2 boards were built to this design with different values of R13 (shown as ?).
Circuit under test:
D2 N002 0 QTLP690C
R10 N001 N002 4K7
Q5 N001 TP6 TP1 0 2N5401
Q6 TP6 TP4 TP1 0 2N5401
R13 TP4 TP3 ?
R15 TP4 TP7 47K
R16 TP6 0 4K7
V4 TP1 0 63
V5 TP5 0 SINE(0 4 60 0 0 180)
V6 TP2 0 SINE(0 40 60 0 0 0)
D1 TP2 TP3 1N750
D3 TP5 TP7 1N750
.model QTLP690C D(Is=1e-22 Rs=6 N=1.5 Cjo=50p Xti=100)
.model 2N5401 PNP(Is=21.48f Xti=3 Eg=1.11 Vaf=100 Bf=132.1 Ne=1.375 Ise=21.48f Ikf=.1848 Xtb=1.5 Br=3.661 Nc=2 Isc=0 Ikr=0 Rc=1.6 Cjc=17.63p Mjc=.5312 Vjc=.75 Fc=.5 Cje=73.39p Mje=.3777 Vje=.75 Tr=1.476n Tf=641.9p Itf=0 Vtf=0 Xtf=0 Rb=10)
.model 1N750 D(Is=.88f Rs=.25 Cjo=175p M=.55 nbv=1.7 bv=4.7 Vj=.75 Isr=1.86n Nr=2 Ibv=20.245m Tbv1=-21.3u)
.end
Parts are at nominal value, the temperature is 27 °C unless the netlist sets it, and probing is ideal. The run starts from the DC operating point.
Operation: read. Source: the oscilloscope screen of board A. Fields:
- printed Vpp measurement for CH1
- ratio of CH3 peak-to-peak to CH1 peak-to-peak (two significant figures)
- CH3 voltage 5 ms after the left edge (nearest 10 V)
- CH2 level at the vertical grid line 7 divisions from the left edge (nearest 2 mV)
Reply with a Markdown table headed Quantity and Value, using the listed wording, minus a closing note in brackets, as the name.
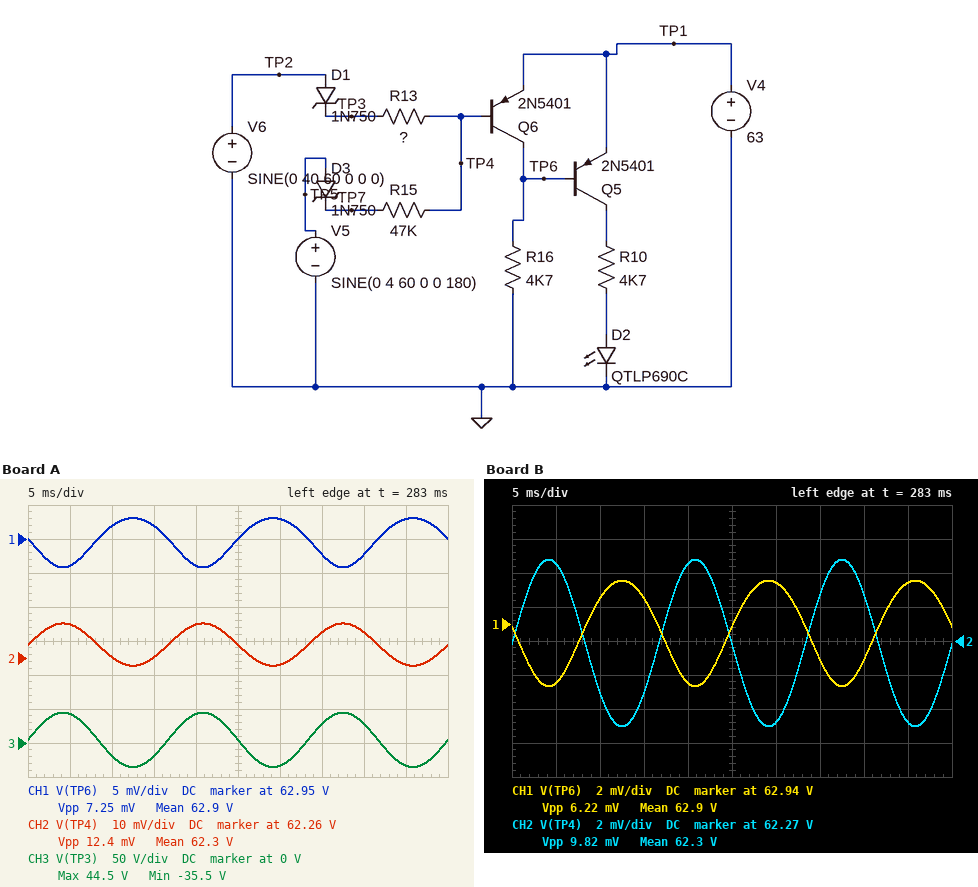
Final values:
| Quantity | Value |
|---|---|
| printed Vpp measurement for CH1 | 7.25 mV |
| ratio of CH3 peak-to-peak to CH1 peak-to-peak | 11000 |
| CH3 voltage 5 ms after the left edge | 40 V |
| CH2 level at the vertical grid line 7 divisions from the left edge | 62.268 V |
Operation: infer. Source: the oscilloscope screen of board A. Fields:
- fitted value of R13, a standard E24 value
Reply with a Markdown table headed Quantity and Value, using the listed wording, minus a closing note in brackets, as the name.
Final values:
| Quantity | Value |
|---|---|
| fitted value of R13, a standard E24 value | 82 kΩ |
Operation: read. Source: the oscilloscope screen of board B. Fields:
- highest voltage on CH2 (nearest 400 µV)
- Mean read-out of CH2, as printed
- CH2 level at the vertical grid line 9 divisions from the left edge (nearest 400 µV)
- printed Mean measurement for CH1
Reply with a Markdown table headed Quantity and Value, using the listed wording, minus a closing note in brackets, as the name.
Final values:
| Quantity | Value |
|---|---|
| highest voltage on CH2 | 62.2708 V |
| Mean read-out of CH2, as printed | 62.3 V |
| CH2 level at the vertical grid line 9 divisions from the left edge | 62.2612 V |
| printed Mean measurement for CH1 | 62.9 V |
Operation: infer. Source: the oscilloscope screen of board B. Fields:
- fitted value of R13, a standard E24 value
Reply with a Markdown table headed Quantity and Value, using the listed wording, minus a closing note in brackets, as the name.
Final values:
| Quantity | Value |
|---|---|
| fitted value of R13, a standard E24 value | 100 kΩ |
